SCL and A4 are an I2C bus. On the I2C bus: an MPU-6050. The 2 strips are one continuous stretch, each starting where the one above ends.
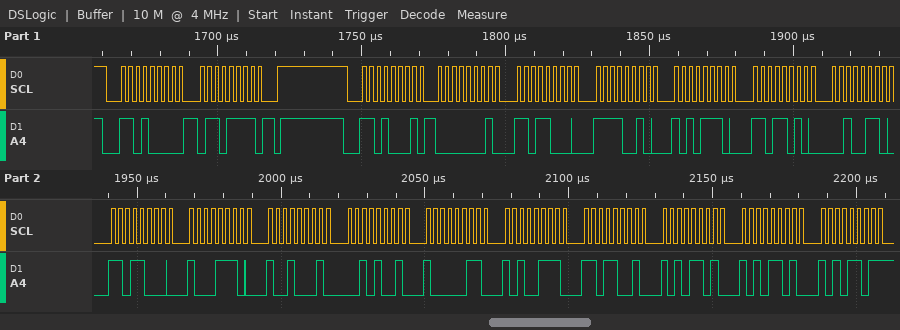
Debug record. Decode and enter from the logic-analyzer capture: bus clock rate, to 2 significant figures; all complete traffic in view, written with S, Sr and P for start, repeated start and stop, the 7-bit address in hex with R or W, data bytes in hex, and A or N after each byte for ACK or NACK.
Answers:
400 kHz
S 68W A 6F A P S 68R A 01 A D8 A F2 A AE A DA A 26 A D8 A 8E A 91 A 29 A 83 A A7 A D9 A AD A AD A AD N
